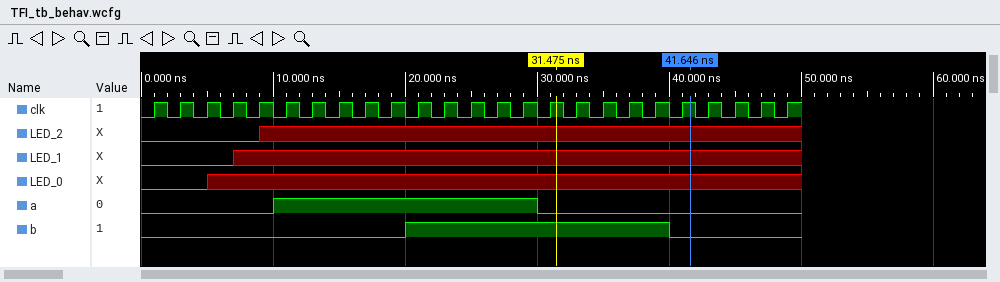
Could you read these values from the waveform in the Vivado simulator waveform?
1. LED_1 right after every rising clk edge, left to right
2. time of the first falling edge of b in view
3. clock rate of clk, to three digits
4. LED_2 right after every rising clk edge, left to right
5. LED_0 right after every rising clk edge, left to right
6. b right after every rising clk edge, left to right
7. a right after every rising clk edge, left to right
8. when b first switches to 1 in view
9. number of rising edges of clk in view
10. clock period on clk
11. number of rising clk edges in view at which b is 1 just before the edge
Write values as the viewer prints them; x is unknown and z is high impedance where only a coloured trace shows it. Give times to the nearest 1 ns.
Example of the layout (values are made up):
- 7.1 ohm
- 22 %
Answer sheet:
- 0 0 0 x x x x x x x x x x x x x x x x x x x x x x
- 40 ns
- 500 MHz
- 0 0 0 0 x x x x x x x x x x x x x x x x x x x x x
- 0 0 x x x x x x x x x x x x x x x x x x x x x x x
- 0 0 0 0 0 0 0 0 0 0 1 1 1 1 1 1 1 1 1 1 0 0 0 0 0
- 0 0 0 0 0 1 1 1 1 1 1 1 1 1 1 0 0 0 0 0 0 0 0 0 0
- 20 ns
- 25
- 2 ns
- 10
